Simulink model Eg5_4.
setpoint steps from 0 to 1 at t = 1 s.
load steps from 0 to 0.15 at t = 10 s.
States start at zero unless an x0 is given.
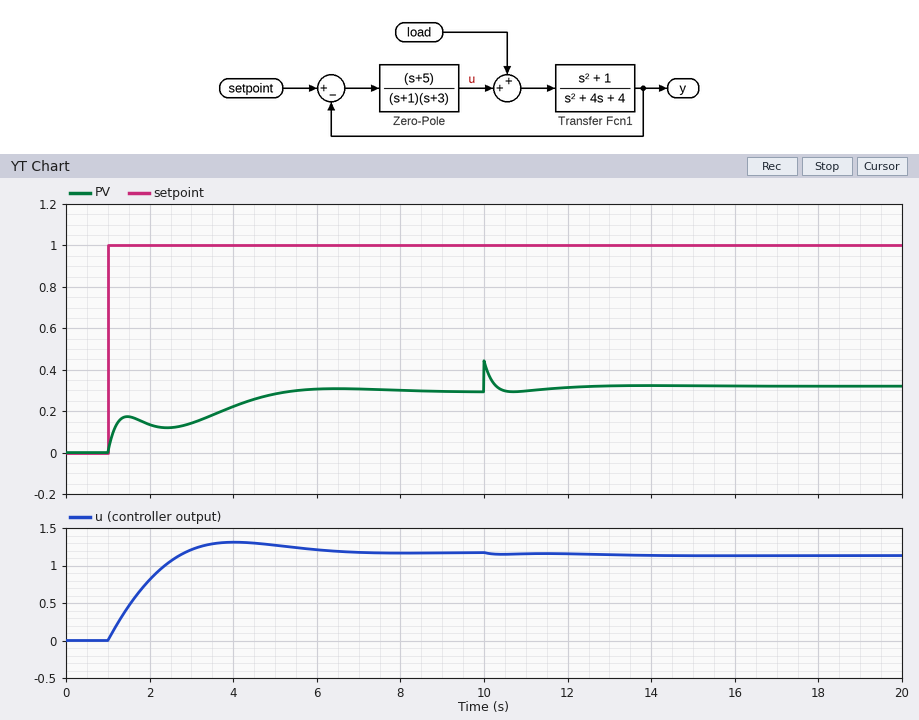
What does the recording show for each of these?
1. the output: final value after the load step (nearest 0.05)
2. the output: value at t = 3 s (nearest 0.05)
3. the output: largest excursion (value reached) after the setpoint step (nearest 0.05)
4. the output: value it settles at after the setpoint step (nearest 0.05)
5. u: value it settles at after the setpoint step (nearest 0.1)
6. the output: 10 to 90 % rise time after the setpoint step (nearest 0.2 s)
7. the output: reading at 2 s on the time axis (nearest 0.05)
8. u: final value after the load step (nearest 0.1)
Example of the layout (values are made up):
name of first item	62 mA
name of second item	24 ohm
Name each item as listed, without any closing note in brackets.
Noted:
the output: final value after the load step	0.30
the output: value at t = 3 s	0.15
the output: largest excursion (value reached) after the setpoint step	0.30
the output: value it settles at after the setpoint step	0.30
u: value it settles at after the setpoint step	1.2
the output: 10 to 90 % rise time after the setpoint step	3.6 s
the output: reading at 2 s on the time axis	0.15
u: final value after the load step	1.1
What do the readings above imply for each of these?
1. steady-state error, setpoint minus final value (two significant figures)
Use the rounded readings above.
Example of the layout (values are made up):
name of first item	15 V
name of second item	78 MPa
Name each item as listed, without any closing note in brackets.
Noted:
steady-state error, setpoint minus final value	0.70
